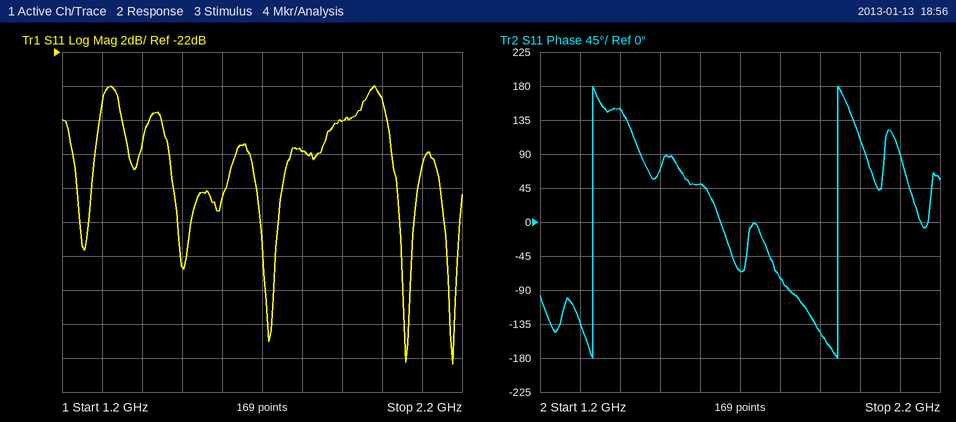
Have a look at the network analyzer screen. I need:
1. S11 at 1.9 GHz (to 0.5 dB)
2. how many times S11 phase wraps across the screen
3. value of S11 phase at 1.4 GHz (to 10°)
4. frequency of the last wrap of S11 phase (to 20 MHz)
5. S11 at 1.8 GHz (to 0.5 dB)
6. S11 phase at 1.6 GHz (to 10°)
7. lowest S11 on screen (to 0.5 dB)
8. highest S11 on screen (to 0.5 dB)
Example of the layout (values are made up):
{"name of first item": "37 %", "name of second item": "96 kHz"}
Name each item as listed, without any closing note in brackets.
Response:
{"S11 at 1.9 GHz": "-26.0 dB", "how many times S11 phase wraps across the screen": "2", "value of S11 phase at 1.4 GHz": "150°", "frequency of the last wrap of S11 phase": "1.94 GHz", "S11 at 1.8 GHz": "-28.0 dB", "S11 phase at 1.6 GHz": "50°", "lowest S11 on screen": "-40.5 dB", "highest S11 on screen": "-24.0 dB"}
